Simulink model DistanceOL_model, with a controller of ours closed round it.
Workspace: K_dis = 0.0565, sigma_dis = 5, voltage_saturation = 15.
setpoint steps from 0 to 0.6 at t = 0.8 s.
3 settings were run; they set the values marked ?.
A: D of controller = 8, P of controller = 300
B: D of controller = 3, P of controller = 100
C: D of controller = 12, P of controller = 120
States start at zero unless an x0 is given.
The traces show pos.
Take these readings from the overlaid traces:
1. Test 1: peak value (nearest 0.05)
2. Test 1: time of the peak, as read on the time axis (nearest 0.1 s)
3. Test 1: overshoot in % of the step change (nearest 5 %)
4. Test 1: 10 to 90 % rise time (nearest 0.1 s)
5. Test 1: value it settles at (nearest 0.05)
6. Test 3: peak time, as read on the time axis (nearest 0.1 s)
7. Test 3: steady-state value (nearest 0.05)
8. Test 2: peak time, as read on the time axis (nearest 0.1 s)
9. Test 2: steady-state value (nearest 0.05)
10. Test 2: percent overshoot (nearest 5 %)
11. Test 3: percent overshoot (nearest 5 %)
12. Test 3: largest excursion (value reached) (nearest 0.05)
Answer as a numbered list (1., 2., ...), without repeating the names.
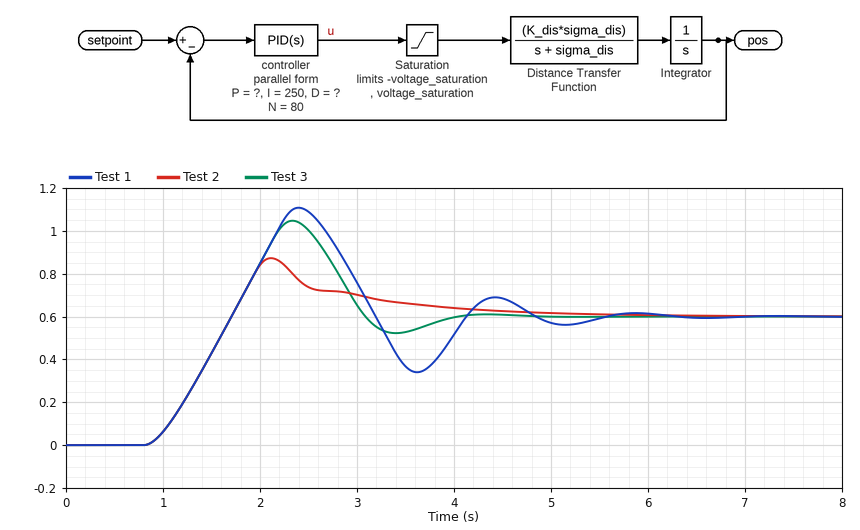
1. 1.10
2. 2.4 s
3. 85 %
4. 0.6 s
5. 0.60
6. 2.3 s
7. 0.60
8. 2.1 s
9. 0.60
10. 45 %
11. 75 %
12. 1.05
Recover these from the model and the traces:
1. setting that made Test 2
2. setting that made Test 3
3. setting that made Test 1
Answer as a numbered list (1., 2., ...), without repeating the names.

1. A
2. C
3. B
